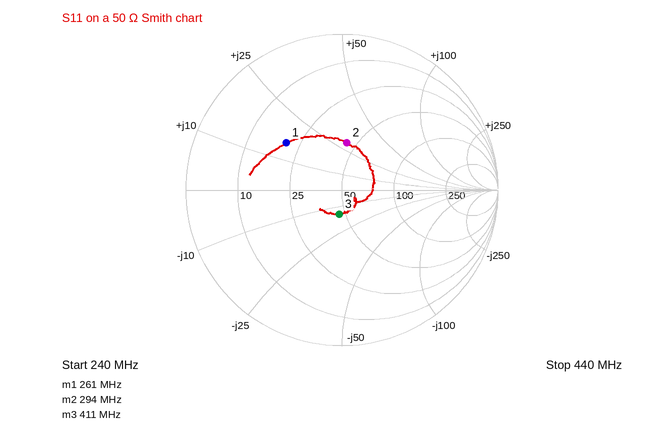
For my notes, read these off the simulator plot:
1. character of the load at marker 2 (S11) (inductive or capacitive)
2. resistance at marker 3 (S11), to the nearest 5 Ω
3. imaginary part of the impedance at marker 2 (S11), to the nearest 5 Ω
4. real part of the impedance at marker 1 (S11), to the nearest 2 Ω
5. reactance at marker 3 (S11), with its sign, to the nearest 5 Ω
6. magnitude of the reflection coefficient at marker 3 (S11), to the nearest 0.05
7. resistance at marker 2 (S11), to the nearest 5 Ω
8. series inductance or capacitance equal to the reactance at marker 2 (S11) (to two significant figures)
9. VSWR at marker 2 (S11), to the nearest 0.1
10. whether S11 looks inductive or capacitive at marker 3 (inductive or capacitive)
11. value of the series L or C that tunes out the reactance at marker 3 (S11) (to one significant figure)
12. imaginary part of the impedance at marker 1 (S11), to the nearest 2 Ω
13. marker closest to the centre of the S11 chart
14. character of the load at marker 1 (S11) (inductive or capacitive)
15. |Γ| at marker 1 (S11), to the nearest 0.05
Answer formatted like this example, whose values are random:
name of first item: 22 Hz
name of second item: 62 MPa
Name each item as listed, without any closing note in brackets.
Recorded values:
character of the load at marker 2 (S11): inductive
resistance at marker 3 (S11), to the nearest 5 Ω: 45 Ω
imaginary part of the impedance at marker 2 (S11), to the nearest 5 Ω: +30 Ω
real part of the impedance at marker 1 (S11), to the nearest 2 Ω: 20 Ω
reactance at marker 3 (S11), with its sign, to the nearest 5 Ω: -15 Ω
magnitude of the reflection coefficient at marker 3 (S11), to the nearest 0.05: 0.15
resistance at marker 2 (S11), to the nearest 5 Ω: 45 Ω
series inductance or capacitance equal to the reactance at marker 2 (S11): 16 nH
VSWR at marker 2 (S11), to the nearest 0.1: 1.9
whether S11 looks inductive or capacitive at marker 3: capacitive
value of the series L or C that tunes out the reactance at marker 3 (S11): 6 nH
imaginary part of the impedance at marker 1 (S11), to the nearest 2 Ω: +16 Ω
marker closest to the centre of the S11 chart: marker 3
character of the load at marker 1 (S11): inductive
|Γ| at marker 1 (S11), to the nearest 0.05: 0.45
